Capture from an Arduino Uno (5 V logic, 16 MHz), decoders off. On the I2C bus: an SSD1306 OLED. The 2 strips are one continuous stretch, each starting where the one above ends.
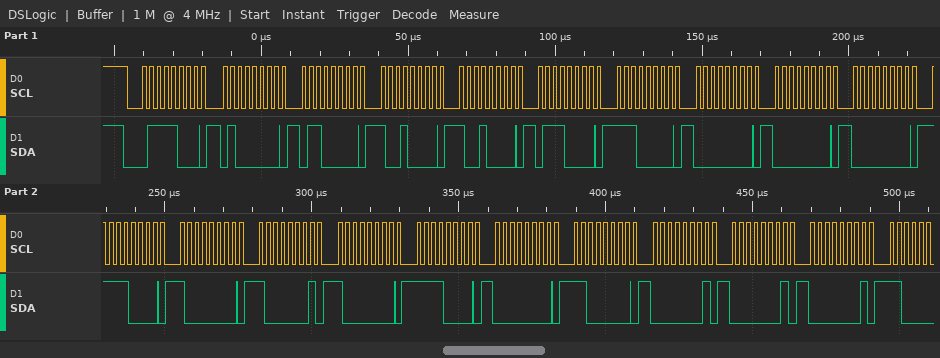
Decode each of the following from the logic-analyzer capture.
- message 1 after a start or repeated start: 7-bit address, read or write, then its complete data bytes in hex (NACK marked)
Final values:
0x3C write: 40 60 90 90 70 E0 00 00 00 F0 80 81 80 F0 00 C0 01 01 01
